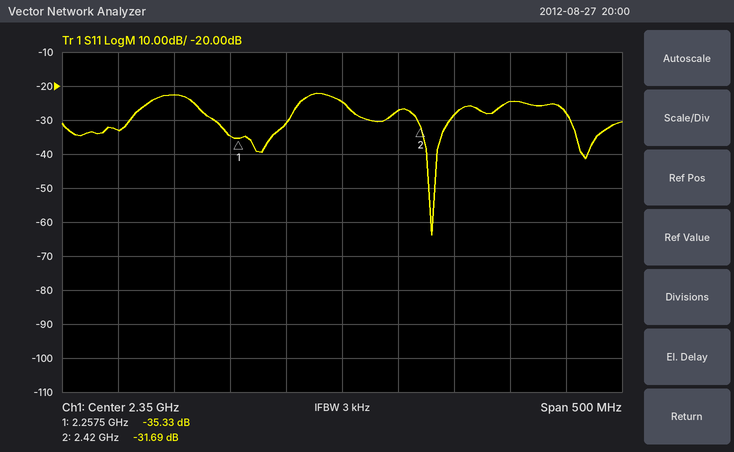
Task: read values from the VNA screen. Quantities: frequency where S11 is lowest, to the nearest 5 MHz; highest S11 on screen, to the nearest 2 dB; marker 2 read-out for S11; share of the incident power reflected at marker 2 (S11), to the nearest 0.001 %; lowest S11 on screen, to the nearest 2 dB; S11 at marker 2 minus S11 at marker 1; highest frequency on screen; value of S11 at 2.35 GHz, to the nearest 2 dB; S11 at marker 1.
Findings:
2.430 GHz
-22 dB
-31.69 dB
0.068 %
-64 dB
3.64 dB
2.6 GHz
-24 dB
-35.33 dB
